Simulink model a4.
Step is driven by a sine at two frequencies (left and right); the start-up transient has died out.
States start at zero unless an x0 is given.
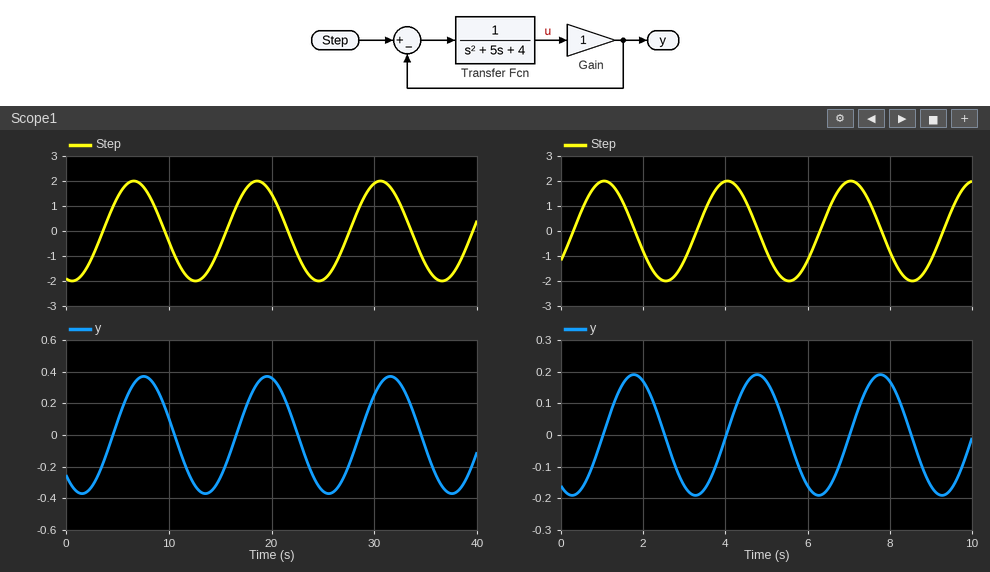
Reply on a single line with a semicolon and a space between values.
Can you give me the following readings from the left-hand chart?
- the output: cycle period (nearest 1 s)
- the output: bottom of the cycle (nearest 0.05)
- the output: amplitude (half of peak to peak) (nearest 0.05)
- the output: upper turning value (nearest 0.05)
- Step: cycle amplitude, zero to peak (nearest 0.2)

12 s; -0.35; 0.35; 0.35; 2.0
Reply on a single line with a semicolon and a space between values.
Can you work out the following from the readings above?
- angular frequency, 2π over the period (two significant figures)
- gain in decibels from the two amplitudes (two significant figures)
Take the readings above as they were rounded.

0.52 rad/s; -15 dB
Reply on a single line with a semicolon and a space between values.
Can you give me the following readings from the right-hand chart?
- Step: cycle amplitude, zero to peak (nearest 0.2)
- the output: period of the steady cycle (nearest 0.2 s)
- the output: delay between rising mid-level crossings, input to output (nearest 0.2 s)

2.0; 3.0 s; 0.8 s
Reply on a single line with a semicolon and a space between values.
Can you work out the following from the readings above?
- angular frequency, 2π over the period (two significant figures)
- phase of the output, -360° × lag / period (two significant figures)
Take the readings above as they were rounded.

2.1 rad/s; -96°
